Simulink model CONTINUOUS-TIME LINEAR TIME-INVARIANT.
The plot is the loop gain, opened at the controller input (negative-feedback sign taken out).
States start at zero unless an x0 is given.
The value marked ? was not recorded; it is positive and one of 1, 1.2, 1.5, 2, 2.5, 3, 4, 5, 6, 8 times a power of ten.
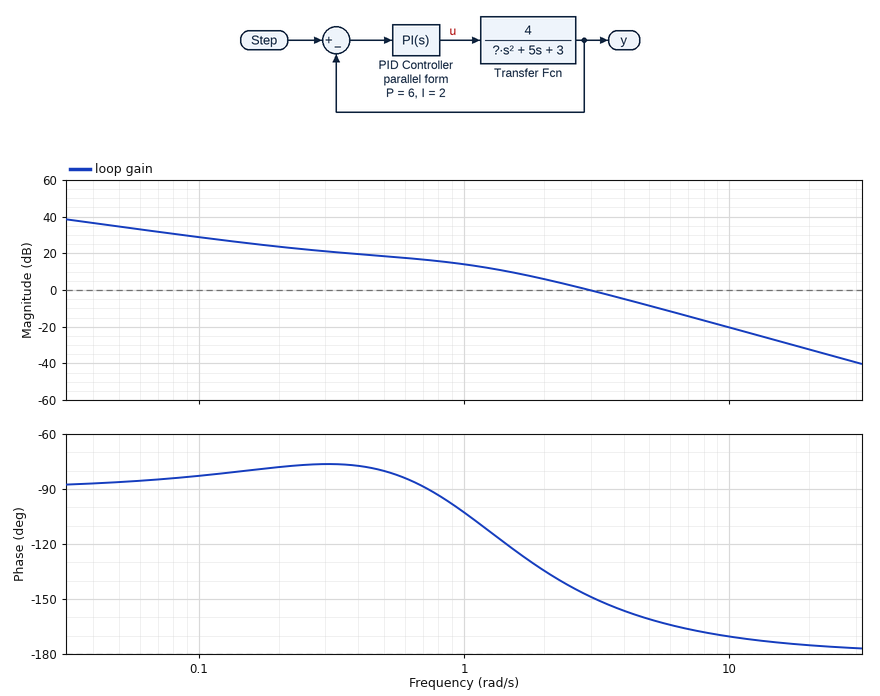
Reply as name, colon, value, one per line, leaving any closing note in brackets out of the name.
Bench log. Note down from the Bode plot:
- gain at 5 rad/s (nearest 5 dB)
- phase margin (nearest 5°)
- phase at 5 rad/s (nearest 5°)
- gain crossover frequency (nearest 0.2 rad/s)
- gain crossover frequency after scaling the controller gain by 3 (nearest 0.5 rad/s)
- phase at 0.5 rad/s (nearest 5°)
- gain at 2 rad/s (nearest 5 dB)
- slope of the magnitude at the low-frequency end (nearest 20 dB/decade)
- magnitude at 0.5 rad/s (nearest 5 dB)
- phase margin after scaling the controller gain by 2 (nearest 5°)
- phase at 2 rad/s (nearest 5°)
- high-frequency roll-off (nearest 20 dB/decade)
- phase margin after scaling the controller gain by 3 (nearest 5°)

gain at 5 rad/s: -10 dB
phase margin: 30°
phase at 5 rad/s: -160°
gain crossover frequency: 3.0 rad/s
gain crossover frequency after scaling the controller gain by 3: 5.5 rad/s
phase at 0.5 rad/s: -80°
gain at 2 rad/s: 5 dB
slope of the magnitude at the low-frequency end: -20 dB/decade
magnitude at 0.5 rad/s: 20 dB
phase margin after scaling the controller gain by 2: 20°
phase at 2 rad/s: -135°
high-frequency roll-off: -40 dB/decade
phase margin after scaling the controller gain by 3: 20°
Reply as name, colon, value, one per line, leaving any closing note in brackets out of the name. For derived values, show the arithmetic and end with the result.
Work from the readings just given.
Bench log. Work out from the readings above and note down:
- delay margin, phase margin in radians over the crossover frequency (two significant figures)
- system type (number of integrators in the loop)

delay margin, phase margin in radians over the crossover frequency: 30 × π / 180 / 3 = 0.17 s
system type: 1
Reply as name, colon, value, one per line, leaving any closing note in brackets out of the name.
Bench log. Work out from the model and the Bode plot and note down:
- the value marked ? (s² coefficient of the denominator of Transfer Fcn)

the value marked ?: 2.5
